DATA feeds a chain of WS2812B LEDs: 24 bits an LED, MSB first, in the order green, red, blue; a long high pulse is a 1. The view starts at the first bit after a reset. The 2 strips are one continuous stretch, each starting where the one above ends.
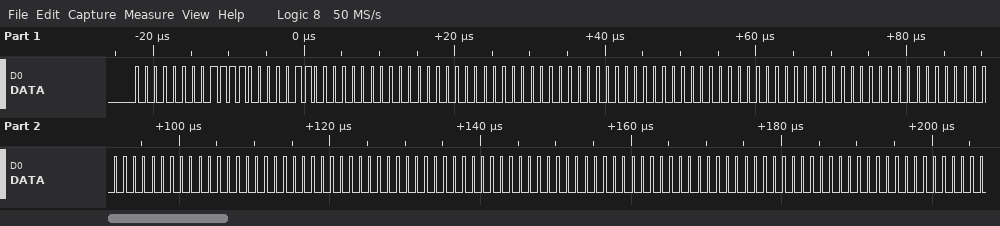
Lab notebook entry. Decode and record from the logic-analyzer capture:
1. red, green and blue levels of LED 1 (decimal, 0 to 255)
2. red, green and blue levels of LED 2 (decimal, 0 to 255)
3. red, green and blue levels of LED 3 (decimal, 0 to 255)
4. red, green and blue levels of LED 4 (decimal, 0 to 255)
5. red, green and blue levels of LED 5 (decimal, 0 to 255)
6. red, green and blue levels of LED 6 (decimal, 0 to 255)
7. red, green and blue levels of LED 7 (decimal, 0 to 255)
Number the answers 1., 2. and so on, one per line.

1. 240, 0, 96
2. 0, 0, 0
3. 0, 0, 0
4. 0, 0, 0
5. 0, 0, 0
6. 0, 0, 0
7. 0, 0, 0
